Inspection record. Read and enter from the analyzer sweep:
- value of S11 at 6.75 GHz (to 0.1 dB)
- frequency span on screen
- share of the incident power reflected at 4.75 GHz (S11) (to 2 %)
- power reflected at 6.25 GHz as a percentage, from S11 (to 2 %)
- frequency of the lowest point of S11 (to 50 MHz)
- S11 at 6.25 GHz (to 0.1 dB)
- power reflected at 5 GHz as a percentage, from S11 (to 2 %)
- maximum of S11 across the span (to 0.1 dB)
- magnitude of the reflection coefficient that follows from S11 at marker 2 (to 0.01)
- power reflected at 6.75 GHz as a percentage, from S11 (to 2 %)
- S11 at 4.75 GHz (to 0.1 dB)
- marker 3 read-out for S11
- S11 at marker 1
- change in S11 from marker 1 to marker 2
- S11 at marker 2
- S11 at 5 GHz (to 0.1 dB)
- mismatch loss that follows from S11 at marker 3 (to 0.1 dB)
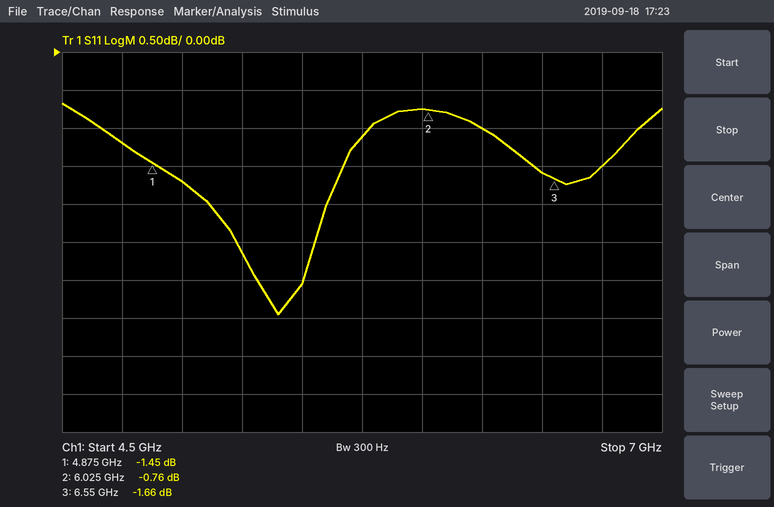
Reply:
-1.5 dB
2.5 GHz
76 %
80 %
5.40 GHz
-1.0 dB
68 %
-0.7 dB
0.92
70 %
-1.2 dB
-1.66 dB
-1.45 dB
0.69 dB
-0.76 dB
-1.7 dB
5.0 dB
